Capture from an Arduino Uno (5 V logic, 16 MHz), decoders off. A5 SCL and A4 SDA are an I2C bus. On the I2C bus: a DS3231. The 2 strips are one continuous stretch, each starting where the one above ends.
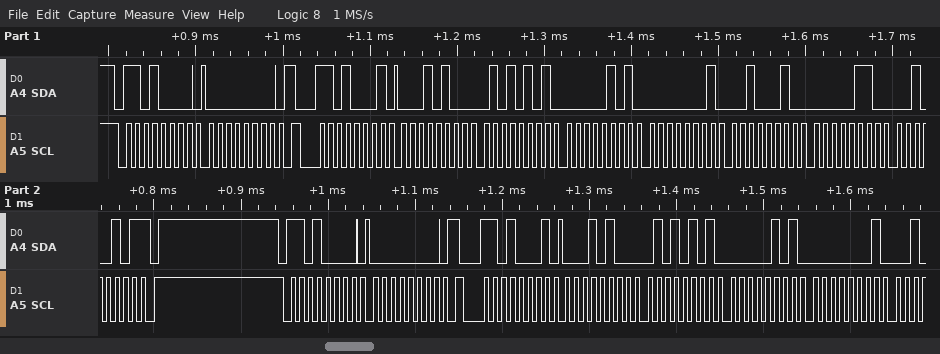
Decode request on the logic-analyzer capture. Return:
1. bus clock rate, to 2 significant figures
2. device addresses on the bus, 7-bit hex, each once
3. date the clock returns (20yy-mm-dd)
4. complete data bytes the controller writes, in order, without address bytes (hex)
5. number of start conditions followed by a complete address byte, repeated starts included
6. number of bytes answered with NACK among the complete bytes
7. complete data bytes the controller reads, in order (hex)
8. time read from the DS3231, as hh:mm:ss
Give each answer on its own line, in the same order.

100 kHz
0x68
2025-06-22
00 00
4
1
14 55 05 01 22 06 25 14 55 05 01
05:55:14
